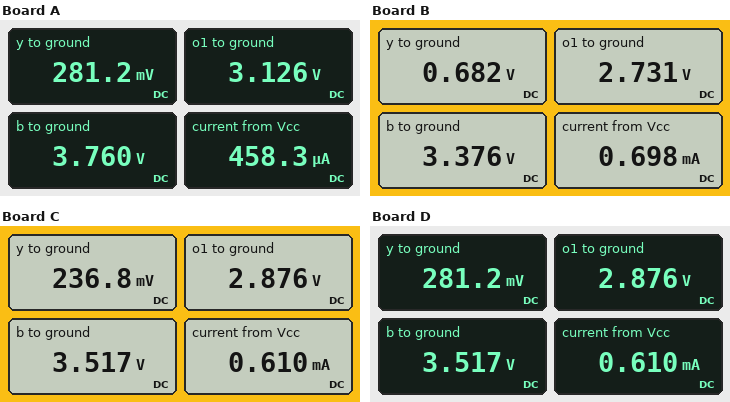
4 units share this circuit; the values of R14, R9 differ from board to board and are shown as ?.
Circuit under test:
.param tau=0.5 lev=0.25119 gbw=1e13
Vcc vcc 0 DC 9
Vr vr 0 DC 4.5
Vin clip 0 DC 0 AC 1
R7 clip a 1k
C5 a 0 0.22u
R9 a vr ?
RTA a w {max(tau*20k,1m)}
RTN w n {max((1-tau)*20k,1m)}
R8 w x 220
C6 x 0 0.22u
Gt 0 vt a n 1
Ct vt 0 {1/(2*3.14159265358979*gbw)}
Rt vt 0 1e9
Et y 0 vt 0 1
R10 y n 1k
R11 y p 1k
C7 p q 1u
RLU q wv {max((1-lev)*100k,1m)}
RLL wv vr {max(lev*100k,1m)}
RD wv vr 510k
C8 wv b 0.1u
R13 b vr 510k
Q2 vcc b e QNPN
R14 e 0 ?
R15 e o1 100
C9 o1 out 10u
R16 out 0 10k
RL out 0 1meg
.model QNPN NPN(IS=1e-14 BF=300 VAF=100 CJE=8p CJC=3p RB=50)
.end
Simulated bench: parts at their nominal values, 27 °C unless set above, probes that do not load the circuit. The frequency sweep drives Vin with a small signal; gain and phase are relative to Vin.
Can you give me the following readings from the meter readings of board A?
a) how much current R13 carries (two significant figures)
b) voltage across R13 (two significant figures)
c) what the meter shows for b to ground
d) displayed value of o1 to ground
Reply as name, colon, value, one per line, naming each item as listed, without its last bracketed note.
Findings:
how much current R13 carries: 1.5 µA
voltage across R13: 740 mV
what the meter shows for b to ground: 3.760 V
displayed value of o1 to ground: 3.126 V
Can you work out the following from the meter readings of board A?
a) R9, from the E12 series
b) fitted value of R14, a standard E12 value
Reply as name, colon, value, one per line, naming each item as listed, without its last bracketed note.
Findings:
R9, from the E12 series: 15 kΩ
fitted value of R14, a standard E12 value: 6.8 kΩ
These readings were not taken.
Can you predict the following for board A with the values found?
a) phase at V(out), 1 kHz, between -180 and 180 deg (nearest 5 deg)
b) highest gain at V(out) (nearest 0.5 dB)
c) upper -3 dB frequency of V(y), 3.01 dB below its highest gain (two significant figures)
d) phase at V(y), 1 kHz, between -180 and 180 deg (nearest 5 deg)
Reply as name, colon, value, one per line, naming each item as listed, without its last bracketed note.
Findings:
phase at V(out), 1 kHz, between -180 and 180 deg: -50 deg
highest gain at V(out): -13.5 dB
upper -3 dB frequency of V(y), 3.01 dB below its highest gain: 840 Hz
phase at V(y), 1 kHz, between -180 and 180 deg: -50 deg
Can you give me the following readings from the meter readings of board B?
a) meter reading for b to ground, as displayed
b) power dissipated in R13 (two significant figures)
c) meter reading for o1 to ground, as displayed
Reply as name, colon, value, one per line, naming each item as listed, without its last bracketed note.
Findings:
meter reading for b to ground, as displayed: 3.376 V
power dissipated in R13: 2.5 µW
meter reading for o1 to ground, as displayed: 2.731 V
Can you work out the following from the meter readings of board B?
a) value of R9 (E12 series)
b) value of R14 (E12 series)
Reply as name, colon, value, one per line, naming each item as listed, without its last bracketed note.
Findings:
value of R9: 5.6 kΩ
value of R14: 3.9 kΩ
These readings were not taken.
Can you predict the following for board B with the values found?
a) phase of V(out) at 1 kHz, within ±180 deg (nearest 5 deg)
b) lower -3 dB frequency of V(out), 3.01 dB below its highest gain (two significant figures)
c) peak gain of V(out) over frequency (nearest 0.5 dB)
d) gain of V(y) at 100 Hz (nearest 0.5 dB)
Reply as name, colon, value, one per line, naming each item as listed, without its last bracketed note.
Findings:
phase of V(out) at 1 kHz, within ±180 deg: -45 deg
lower -3 dB frequency of V(out), 3.01 dB below its highest gain: 5.6 Hz
peak gain of V(out) over frequency: -14.5 dB
gain of V(y) at 100 Hz: -1.5 dB
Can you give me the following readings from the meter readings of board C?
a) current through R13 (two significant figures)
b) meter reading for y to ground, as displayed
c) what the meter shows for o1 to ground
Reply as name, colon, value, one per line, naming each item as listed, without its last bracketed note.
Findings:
current through R13: 1.9 µA
meter reading for y to ground, as displayed: 236.8 mV
what the meter shows for o1 to ground: 2.876 V
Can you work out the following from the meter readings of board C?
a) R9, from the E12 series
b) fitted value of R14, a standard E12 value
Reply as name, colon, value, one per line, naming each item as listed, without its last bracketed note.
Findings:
R9, from the E12 series: 18 kΩ
fitted value of R14, a standard E12 value: 4.7 kΩ
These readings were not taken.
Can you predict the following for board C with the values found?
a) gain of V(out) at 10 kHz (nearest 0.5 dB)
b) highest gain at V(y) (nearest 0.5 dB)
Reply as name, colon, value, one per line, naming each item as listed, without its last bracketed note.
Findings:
gain of V(out) at 10 kHz: -35.0 dB
highest gain at V(y): -0.5 dB
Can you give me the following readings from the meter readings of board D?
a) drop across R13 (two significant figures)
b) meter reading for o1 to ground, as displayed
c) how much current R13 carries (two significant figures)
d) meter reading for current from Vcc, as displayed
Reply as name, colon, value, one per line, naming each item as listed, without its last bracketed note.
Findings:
drop across R13: 980 mV
meter reading for o1 to ground, as displayed: 2.876 V
how much current R13 carries: 1.9 µA
meter reading for current from Vcc, as displayed: 0.610 mA
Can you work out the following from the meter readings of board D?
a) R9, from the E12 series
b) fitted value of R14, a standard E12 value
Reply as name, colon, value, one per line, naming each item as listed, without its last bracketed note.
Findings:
R9, from the E12 series: 15 kΩ
fitted value of R14, a standard E12 value: 4.7 kΩ
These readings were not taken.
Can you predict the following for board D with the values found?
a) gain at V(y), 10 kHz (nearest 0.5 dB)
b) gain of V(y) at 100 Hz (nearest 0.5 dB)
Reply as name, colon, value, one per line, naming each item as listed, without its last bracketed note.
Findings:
gain at V(y), 10 kHz: -22.0 dB
gain of V(y) at 100 Hz: -0.5 dB
